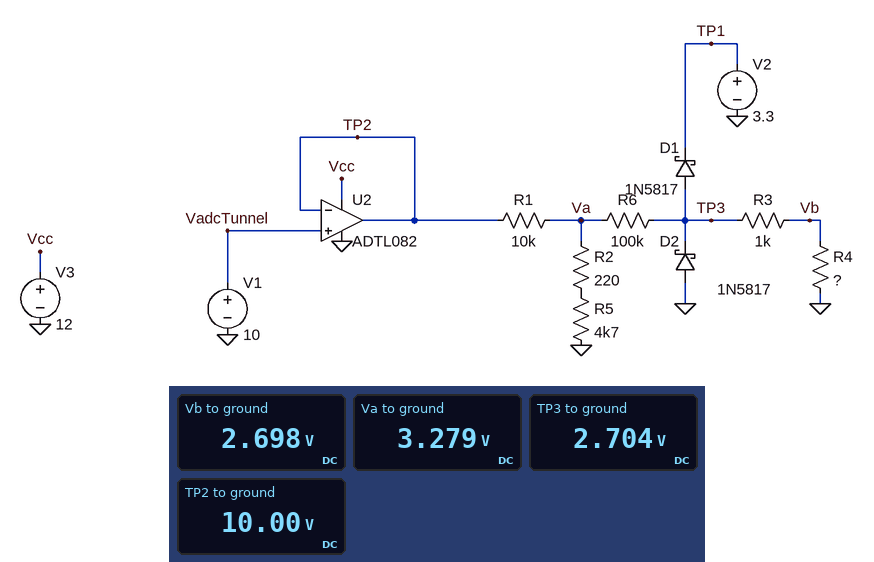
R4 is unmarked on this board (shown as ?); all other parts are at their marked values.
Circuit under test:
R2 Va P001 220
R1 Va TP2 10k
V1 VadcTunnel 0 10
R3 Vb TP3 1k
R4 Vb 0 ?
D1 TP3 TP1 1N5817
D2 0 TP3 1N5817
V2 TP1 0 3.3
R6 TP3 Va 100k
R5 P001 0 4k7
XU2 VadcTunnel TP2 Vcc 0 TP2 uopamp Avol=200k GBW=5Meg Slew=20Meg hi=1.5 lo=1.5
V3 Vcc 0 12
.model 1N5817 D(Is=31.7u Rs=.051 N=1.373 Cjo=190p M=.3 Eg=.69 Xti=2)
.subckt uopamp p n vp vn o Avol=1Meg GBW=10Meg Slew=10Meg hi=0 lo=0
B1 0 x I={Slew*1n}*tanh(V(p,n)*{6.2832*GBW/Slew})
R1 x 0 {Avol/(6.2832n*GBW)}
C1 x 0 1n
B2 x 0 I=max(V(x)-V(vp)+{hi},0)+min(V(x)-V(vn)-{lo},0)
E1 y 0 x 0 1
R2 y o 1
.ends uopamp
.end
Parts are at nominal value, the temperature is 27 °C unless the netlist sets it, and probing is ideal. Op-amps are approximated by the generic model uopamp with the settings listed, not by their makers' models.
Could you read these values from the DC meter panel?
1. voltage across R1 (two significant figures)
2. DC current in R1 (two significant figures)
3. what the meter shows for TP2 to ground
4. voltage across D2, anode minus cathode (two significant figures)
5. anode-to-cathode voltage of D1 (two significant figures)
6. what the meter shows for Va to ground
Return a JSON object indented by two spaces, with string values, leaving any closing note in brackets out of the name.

{
  "voltage across R1": "6.7 V",
  "DC current in R1": "670 µA",
  "what the meter shows for TP2 to ground": "10.00 V",
  "voltage across D2, anode minus cathode": "-2.7 V",
  "anode-to-cathode voltage of D1": "-600 mV",
  "what the meter shows for Va to ground": "3.279 V"
}
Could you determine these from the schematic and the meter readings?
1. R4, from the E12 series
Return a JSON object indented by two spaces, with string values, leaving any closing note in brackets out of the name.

{
  "R4, from the E12 series": "470 kΩ"
}
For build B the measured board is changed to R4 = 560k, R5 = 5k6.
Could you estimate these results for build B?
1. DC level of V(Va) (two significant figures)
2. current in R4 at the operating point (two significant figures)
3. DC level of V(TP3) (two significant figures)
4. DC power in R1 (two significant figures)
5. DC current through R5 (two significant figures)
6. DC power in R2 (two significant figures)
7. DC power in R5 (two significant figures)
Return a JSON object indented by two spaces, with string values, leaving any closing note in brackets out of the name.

{
  "DC level of V(Va)": "3.7 V",
  "current in R4 at the operating point": "5.5 µA",
  "DC level of V(TP3)": "3.1 V",
  "DC power in R1": "4.0 mW",
  "DC current through R5": "630 µA",
  "DC power in R2": "87 µW",
  "DC power in R5": "2.2 mW"
}
